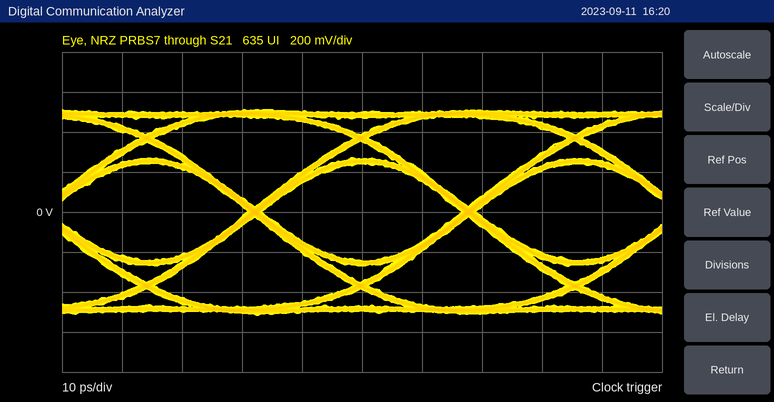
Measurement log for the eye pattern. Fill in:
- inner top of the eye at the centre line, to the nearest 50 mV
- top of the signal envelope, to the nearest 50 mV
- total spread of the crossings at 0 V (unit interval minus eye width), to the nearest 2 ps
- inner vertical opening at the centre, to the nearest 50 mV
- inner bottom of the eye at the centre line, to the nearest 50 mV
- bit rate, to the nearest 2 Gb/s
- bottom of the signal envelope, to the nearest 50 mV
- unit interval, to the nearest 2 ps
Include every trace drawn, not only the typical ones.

250 mV
500 mV
2 ps
500 mV
-250 mV
28 Gb/s
-500 mV
36 ps
